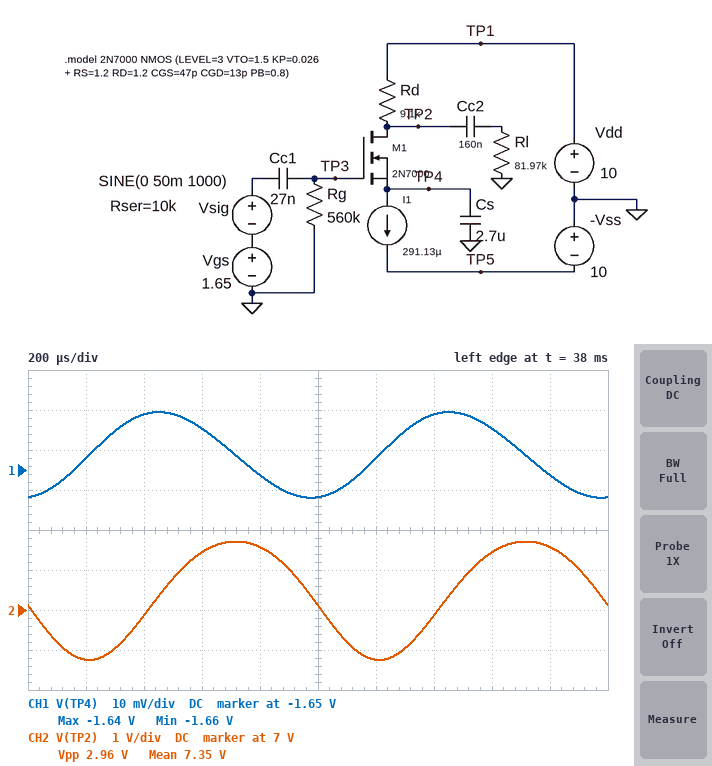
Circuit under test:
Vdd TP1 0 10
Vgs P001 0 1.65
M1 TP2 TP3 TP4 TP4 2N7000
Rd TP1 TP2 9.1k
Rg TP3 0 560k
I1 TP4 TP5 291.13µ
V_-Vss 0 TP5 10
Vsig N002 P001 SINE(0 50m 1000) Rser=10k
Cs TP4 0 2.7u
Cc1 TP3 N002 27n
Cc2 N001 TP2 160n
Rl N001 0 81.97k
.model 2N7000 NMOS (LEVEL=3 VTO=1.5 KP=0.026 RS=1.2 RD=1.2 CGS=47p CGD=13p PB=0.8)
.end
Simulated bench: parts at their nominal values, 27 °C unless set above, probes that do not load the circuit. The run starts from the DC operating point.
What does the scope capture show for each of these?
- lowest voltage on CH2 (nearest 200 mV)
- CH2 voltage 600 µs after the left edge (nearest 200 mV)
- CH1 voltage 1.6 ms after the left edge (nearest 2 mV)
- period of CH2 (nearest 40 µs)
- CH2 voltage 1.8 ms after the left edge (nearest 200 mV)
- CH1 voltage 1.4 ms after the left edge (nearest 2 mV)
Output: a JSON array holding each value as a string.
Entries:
["5.8 V", "8.4 V", "-1.640 V", "1.00 ms", "8.6 V", "-1.636 V"]
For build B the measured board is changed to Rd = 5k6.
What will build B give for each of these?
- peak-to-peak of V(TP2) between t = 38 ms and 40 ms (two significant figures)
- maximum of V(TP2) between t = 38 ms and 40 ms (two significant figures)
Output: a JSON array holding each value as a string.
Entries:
["1.9 V", "9.2 V"]
